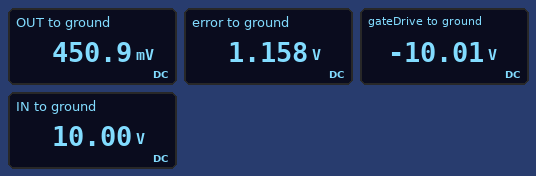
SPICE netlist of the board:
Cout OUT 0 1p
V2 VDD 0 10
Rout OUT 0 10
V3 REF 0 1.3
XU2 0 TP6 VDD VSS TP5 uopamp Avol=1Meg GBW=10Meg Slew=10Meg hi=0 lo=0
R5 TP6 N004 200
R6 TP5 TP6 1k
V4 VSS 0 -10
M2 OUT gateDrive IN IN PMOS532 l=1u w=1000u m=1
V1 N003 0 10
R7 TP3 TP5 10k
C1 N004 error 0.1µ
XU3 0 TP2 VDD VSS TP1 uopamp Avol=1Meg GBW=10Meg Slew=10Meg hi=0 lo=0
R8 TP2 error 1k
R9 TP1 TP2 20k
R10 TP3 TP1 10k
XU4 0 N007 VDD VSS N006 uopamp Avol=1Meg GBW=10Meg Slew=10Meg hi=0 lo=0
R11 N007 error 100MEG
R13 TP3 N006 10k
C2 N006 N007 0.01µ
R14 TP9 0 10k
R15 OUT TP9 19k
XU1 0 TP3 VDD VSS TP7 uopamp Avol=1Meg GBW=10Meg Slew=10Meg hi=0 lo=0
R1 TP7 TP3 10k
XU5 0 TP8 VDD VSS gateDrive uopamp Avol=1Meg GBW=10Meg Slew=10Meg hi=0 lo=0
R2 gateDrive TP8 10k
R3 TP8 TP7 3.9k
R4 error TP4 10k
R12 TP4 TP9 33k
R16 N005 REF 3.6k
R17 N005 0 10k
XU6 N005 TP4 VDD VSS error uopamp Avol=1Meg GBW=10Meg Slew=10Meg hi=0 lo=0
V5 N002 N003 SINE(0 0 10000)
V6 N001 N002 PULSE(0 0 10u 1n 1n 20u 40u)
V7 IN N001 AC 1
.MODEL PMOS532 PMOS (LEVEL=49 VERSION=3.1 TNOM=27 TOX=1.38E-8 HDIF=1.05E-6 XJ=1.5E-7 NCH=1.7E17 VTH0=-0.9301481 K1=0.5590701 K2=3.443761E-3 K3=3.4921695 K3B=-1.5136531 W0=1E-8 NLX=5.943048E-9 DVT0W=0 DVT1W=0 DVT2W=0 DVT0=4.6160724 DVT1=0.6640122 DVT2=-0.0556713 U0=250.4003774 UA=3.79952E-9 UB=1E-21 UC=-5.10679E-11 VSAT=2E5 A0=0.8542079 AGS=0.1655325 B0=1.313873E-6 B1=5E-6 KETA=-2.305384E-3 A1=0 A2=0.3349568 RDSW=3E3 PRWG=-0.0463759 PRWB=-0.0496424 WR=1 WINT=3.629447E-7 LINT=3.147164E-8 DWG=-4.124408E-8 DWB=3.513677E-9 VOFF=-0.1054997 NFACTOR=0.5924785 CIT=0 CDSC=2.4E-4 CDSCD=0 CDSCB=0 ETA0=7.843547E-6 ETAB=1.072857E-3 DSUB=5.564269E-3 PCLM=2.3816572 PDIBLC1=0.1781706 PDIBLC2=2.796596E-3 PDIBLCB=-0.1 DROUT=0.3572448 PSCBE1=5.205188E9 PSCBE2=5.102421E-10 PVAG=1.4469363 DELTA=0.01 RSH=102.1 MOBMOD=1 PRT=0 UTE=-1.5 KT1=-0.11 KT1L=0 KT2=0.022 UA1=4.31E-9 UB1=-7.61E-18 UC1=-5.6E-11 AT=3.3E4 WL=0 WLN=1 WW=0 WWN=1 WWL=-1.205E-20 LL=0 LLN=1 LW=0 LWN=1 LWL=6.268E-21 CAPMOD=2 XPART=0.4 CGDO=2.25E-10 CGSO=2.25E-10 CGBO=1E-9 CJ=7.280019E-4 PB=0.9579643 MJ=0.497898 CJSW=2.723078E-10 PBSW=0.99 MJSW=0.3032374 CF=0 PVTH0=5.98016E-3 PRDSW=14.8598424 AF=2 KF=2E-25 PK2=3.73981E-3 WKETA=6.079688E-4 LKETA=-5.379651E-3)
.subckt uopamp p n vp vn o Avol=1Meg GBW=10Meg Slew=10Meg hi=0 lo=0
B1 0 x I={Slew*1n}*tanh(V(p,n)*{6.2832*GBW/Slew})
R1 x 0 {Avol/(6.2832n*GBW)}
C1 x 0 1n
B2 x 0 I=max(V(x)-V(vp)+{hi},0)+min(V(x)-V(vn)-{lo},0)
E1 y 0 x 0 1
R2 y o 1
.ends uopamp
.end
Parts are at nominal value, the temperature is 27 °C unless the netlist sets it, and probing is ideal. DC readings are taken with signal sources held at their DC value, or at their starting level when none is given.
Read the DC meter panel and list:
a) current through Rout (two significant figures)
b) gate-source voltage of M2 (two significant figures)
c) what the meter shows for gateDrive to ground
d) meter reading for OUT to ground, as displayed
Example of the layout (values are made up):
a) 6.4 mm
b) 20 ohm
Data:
a) 45 mA
b) -20 V
c) -10.01 V
d) 450.9 mV
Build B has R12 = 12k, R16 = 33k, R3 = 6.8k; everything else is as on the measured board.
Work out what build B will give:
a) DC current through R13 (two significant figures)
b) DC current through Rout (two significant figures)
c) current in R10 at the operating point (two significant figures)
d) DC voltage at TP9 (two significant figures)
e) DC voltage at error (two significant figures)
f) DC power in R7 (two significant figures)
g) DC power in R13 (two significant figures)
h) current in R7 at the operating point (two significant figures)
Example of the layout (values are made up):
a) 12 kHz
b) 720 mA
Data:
a) 810 µA
b) 45 mA
c) 570 µA
d) 210 mV
e) 380 mV
f) 360 µW
g) 6.6 mW
h) 190 µA
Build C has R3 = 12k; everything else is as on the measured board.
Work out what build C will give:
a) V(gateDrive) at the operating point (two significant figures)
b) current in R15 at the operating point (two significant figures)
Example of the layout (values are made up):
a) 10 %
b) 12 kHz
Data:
a) -8.3 V
b) 8.5 µA
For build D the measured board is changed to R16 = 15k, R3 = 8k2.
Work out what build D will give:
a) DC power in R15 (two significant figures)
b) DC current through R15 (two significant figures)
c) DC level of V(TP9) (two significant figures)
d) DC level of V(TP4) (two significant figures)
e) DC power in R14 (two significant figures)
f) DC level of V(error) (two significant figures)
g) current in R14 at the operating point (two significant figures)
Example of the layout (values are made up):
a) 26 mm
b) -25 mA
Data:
a) 2.9 µW
b) 12 µA
c) 220 mV
d) 520 mV
e) 4.7 µW
f) 610 mV
g) 22 µA
